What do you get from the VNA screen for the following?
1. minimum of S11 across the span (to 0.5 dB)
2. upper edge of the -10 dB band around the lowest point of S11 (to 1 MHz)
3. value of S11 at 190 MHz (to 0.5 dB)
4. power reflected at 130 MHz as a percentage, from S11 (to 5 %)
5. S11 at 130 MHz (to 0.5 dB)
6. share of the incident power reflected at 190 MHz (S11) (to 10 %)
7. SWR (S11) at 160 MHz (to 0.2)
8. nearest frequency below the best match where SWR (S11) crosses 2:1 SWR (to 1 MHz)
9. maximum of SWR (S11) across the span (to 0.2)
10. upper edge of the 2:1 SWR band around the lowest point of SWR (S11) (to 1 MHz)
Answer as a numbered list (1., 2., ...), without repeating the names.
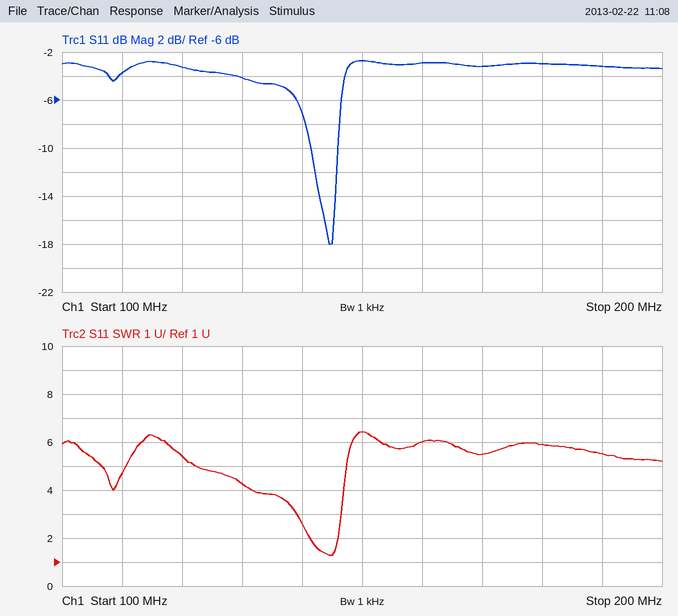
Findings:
1. -18.0 dB
2. 146 MHz
3. -3.0 dB
4. 40 %
5. -4.0 dB
6. 50 %
7. 6.0
8. 141 MHz
9. 6.4
10. 146 MHz
